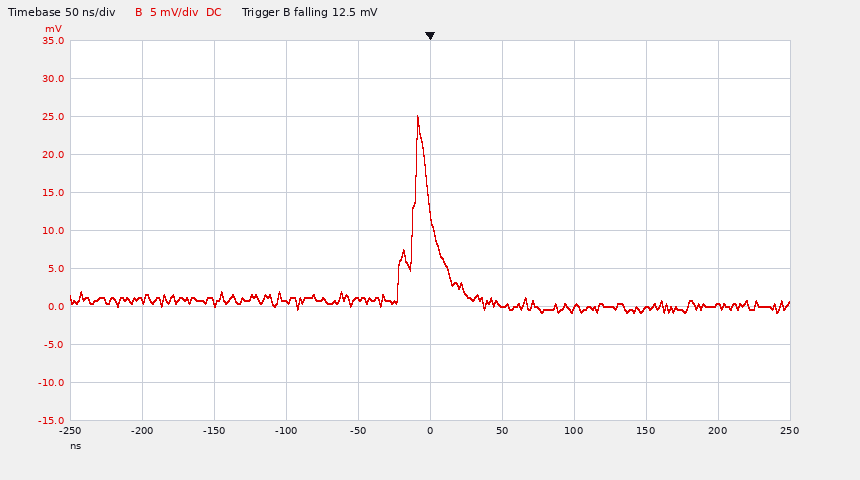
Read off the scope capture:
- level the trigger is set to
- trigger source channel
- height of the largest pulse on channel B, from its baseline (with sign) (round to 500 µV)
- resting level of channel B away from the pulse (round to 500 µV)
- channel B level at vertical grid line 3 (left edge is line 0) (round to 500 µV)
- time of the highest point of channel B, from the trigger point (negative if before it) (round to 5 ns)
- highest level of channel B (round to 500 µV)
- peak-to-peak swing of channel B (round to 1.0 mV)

12.5 mV
channel B
+24.5 mV
500 µV
500 µV
-10 ns
25.0 mV
26.0 mV
